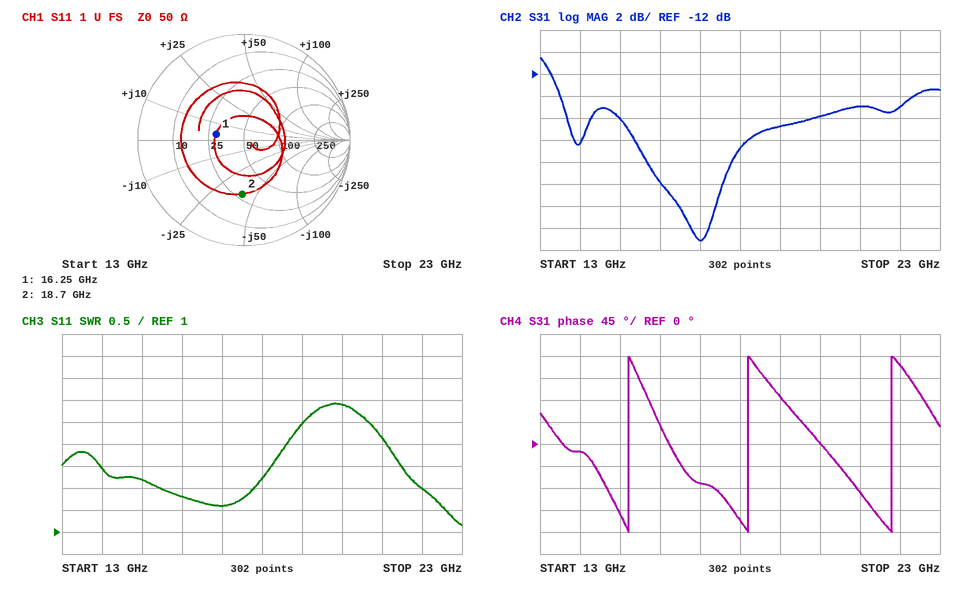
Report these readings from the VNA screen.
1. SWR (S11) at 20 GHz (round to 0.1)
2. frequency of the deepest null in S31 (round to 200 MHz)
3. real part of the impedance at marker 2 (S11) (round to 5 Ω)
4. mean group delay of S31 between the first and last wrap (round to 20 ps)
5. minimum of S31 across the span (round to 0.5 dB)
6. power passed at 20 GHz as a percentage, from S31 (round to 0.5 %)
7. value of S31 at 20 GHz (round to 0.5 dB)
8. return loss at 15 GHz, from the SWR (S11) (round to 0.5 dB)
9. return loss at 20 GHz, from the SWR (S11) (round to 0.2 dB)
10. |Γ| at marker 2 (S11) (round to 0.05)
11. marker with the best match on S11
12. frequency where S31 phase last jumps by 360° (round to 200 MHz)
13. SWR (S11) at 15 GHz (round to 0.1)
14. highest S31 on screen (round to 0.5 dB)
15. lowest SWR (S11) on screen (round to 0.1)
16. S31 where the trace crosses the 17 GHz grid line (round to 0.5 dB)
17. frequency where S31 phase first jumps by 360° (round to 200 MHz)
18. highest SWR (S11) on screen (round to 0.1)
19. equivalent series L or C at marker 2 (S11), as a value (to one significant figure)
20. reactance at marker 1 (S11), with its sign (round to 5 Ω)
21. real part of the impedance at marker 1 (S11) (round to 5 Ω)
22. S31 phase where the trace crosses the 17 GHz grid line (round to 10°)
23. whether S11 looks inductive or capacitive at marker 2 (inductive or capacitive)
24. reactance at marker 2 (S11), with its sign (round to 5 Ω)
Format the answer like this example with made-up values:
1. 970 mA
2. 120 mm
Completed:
1. 3.9
2. 17.0 GHz
3. 30 Ω
4. 300 ps
5. -27.0 dB
6. 2.5 %
7. -16.0 dB
8. 8.5 dB
9. 4.6 dB
10. 0.50
11. marker 1
12. 21.8 GHz
13. 2.2
14. -10.5 dB
15. 1.2
16. -27.0 dB
17. 15.2 GHz
18. 3.9
19. 200 fF
20. +5 Ω
21. 30 Ω
22. -80°
23. capacitive
24. -40 Ω
